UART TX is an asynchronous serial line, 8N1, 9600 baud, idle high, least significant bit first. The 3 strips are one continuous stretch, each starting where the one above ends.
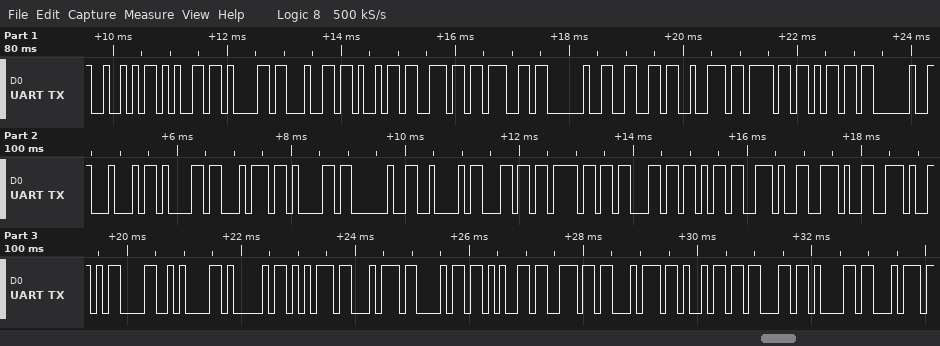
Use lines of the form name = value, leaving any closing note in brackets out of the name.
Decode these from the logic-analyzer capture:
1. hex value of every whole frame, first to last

hex value of every whole frame, first to last = 52 65 61 64 69 6E 67 20 66 72 6F 6D 20 44 61 74 61 20 42 6C 6F 63 6B 2E 2E 2E 0D 0A 41 75 74 68 65 6E 74 69 63 61 74
